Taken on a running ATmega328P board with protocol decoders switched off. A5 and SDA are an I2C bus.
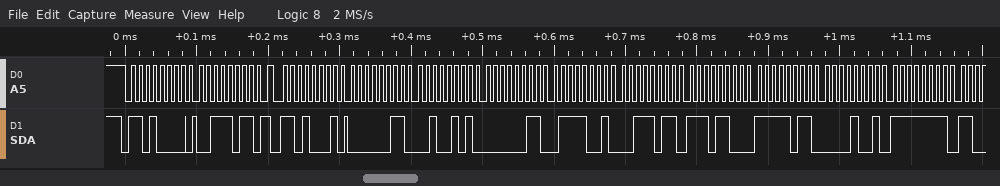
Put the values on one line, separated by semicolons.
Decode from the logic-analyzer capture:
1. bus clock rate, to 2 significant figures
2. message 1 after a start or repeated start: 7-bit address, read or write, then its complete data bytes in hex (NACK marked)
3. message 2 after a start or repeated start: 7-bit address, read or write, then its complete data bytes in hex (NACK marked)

100 kHz; 0x68 write: 3B; 0x68 read: 03 25 03 79 3B EC FB 09 FF
